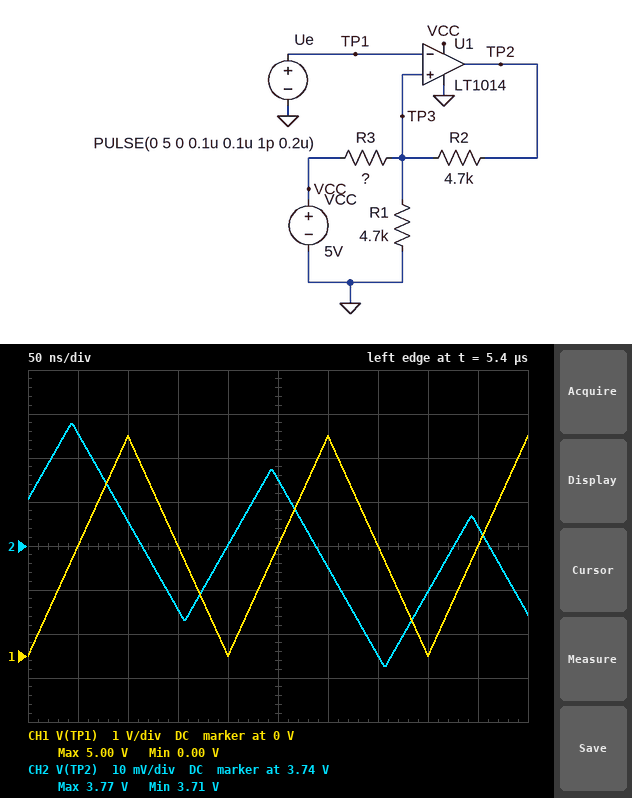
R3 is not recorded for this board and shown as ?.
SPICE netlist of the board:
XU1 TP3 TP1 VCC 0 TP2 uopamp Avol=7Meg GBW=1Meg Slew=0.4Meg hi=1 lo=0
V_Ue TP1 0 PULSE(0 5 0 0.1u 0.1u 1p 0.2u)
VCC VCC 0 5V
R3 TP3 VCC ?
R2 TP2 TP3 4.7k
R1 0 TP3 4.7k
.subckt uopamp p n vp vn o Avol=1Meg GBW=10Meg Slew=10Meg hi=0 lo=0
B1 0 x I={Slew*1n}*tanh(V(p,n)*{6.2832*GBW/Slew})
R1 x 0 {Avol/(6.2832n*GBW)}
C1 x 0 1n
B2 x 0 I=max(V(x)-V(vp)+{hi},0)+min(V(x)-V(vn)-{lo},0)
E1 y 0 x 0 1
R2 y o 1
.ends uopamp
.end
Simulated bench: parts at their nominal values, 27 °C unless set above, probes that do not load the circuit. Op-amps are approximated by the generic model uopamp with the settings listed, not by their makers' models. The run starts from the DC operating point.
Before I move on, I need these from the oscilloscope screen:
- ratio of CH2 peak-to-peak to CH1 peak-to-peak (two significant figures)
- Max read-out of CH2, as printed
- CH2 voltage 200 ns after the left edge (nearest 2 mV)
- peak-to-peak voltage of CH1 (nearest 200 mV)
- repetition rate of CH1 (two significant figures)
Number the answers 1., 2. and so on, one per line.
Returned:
1. 0.011
2. 3.77 V
3. 3.740 V
4. 5.0 V
5. 5.0 MHz
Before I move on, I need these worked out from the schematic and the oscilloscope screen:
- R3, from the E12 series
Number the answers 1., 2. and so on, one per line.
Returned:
1. 22 kΩ
